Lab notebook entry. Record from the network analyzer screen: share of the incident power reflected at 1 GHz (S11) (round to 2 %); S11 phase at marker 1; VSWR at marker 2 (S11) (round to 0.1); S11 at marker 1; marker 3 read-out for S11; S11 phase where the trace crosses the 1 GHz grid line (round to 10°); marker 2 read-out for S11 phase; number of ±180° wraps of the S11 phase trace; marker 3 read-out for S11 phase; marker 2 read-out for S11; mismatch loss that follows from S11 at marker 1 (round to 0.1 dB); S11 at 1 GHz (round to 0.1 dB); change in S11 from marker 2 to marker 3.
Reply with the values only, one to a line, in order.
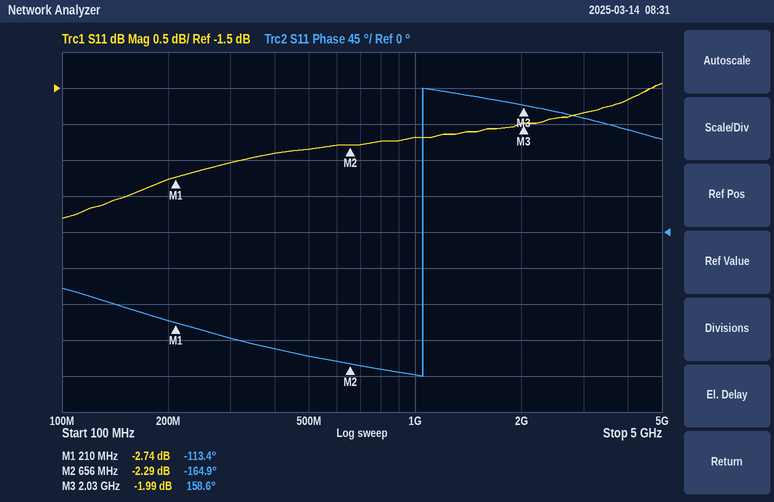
60 %
-113.4°
7.6
-2.74 dB
-1.99 dB
-180°
-164.9°
1
158.6°
-2.29 dB
3.3 dB
-2.2 dB
0.30 dB
